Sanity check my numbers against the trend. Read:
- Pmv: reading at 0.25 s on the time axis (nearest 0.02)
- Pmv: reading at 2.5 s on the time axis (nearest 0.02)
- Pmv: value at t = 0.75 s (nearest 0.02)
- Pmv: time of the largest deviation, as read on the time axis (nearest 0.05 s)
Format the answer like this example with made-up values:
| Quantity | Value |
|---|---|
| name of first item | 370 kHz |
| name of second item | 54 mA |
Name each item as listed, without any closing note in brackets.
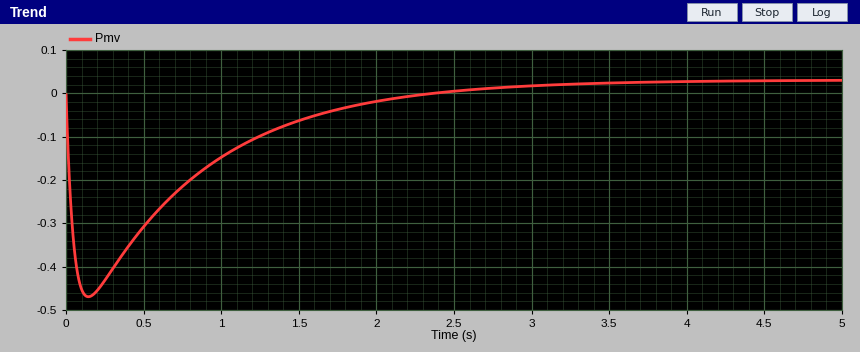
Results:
| Quantity | Value |
|---|---|
| Pmv: reading at 0.25 s on the time axis | -0.44 |
| Pmv: reading at 2.5 s on the time axis | 0.00 |
| Pmv: value at t = 0.75 s | -0.22 |
| Pmv: time of the largest deviation, as read on the time axis | 0.15 s |
